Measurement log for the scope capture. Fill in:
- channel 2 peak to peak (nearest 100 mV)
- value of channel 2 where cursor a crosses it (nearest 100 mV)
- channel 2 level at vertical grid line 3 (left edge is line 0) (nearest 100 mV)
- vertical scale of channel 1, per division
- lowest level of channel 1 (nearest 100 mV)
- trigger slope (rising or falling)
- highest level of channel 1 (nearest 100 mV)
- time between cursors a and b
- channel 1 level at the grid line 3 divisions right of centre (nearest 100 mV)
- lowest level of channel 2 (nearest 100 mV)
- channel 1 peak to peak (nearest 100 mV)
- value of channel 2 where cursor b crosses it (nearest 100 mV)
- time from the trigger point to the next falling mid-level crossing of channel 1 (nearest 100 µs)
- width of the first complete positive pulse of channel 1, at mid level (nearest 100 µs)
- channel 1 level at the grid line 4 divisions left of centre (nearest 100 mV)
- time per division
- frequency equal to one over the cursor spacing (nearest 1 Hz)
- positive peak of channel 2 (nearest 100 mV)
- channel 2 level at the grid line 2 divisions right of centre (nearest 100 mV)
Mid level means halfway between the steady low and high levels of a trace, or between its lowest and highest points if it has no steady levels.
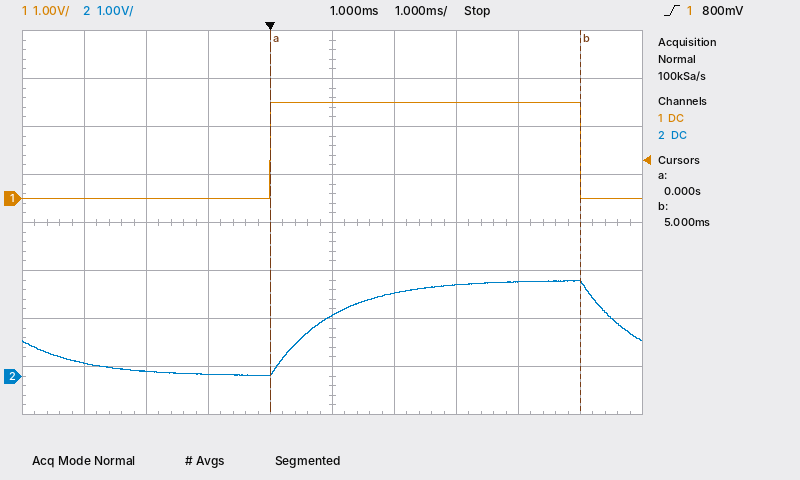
2.0 V
100 mV
0.0 V
1 V
0.0 V
rising
2.0 V
5.0 ms
2.0 V
0.0 V
2.0 V
1.9 V
5.0 ms
5.0 ms
0.0 V
1 ms
200 Hz
2.0 V
1.9 V
